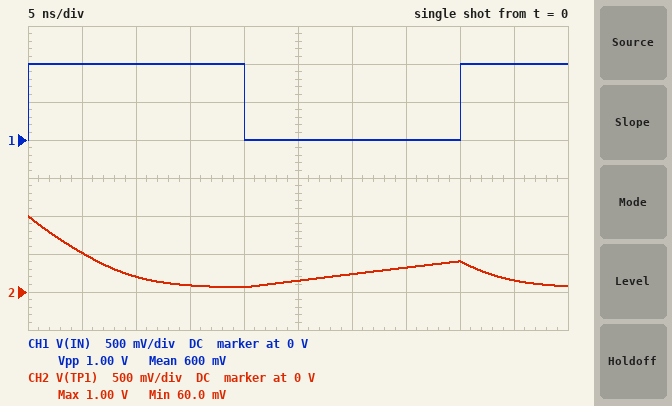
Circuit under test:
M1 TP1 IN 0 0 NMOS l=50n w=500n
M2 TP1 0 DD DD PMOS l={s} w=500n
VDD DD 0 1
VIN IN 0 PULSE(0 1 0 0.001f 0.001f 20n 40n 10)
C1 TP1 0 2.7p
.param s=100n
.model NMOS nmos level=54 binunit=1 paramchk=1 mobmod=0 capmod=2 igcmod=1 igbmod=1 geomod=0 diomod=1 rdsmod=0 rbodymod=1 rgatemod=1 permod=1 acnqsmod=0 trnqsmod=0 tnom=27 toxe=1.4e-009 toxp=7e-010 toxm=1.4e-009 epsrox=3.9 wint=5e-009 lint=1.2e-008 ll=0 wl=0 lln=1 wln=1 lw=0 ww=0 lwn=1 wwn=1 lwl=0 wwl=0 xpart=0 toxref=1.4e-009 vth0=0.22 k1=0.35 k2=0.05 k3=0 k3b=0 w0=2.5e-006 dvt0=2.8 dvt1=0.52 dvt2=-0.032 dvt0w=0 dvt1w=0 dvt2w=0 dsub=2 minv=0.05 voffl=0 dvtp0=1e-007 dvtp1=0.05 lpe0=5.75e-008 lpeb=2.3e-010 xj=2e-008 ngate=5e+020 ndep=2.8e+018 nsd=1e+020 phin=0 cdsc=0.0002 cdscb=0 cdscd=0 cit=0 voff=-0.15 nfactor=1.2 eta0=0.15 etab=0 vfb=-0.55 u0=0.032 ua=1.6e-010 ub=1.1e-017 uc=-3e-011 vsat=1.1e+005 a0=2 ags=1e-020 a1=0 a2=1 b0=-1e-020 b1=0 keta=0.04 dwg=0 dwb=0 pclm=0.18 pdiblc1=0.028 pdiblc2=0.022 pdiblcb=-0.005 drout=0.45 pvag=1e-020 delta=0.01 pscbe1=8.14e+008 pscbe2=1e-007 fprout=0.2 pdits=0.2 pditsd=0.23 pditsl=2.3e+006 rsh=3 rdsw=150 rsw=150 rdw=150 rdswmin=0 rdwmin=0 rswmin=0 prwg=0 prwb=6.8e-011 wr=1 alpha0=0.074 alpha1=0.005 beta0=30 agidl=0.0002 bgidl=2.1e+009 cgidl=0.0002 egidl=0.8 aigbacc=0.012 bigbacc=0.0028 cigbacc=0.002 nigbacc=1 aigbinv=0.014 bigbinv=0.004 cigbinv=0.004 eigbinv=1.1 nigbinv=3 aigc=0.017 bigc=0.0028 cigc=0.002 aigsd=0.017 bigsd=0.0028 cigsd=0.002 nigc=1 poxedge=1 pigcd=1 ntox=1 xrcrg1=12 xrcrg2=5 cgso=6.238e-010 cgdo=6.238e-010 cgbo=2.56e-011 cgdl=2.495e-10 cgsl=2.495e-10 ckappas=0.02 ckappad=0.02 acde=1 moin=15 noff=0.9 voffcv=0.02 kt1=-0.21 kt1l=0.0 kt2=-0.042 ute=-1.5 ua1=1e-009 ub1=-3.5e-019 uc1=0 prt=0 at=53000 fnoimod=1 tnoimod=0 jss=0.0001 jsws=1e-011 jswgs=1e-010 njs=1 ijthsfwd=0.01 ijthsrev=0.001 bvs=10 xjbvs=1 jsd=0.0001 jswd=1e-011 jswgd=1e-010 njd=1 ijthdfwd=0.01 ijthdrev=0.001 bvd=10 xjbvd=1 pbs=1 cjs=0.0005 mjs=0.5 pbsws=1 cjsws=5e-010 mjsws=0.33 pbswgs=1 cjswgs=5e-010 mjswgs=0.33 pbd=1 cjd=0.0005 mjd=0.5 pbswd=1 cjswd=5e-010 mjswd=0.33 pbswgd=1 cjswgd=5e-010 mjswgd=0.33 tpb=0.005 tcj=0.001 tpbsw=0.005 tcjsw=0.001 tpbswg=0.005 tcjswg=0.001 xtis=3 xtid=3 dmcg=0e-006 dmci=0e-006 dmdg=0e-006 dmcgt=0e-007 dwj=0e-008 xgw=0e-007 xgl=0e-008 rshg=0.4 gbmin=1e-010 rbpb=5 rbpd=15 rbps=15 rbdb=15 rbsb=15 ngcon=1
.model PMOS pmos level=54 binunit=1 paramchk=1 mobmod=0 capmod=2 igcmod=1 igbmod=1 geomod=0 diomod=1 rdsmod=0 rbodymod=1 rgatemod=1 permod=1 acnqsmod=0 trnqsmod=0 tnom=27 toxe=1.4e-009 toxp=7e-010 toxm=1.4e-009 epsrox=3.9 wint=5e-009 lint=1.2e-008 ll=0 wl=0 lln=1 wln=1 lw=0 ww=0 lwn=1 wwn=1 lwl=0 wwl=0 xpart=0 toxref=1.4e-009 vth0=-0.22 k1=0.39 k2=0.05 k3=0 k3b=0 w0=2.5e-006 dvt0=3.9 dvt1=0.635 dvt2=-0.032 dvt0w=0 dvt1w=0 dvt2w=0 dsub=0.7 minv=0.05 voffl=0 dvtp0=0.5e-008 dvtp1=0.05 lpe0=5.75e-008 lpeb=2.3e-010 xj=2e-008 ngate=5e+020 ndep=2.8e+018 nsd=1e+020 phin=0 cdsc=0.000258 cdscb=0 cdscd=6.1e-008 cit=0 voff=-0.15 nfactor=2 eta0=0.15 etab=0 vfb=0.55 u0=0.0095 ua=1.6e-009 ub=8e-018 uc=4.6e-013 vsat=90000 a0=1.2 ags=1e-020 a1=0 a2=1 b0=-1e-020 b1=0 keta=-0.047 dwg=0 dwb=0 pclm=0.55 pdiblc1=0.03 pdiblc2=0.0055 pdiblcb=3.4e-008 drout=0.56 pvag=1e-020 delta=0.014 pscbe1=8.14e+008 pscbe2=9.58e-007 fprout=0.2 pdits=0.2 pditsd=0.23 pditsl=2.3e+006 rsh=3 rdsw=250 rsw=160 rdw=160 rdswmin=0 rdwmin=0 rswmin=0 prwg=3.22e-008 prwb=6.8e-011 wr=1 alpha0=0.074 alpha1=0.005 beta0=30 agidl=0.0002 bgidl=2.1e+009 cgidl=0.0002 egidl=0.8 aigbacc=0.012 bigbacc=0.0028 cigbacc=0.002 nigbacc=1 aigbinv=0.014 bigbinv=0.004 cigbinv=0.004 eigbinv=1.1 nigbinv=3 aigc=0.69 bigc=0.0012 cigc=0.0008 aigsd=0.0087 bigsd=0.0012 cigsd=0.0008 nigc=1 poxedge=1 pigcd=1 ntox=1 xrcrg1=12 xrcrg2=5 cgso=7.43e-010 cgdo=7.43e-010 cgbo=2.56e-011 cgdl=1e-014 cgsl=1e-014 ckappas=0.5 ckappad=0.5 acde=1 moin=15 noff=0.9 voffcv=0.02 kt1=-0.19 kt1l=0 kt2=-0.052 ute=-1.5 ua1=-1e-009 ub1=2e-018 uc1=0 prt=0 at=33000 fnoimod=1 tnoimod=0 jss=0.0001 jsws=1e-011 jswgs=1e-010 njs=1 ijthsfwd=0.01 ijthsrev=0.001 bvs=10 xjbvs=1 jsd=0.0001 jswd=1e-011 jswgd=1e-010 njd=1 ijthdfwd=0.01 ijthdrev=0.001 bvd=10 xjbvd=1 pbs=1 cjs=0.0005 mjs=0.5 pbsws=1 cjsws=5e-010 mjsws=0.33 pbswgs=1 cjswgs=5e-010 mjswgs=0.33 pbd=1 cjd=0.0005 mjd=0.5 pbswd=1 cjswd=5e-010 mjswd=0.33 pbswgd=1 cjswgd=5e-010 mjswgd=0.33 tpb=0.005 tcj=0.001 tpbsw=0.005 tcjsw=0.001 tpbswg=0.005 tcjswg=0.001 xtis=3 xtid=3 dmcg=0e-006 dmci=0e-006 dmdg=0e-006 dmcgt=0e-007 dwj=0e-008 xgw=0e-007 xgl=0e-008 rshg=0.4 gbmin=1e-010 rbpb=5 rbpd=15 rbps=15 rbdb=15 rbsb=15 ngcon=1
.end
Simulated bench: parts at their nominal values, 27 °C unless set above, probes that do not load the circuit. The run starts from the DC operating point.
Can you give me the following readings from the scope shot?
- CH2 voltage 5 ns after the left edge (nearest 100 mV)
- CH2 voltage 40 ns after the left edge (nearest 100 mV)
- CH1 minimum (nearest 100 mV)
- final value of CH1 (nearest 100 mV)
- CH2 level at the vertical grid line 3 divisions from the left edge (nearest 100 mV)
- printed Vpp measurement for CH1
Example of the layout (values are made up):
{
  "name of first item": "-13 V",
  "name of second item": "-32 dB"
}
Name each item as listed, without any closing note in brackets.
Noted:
{
  "CH2 voltage 5 ns after the left edge": "500 mV",
  "CH2 voltage 40 ns after the left edge": "400 mV",
  "CH1 minimum": "0 V",
  "final value of CH1": "1.0 V",
  "CH2 level at the vertical grid line 3 divisions from the left edge": "100 mV",
  "printed Vpp measurement for CH1": "1.00 V"
}
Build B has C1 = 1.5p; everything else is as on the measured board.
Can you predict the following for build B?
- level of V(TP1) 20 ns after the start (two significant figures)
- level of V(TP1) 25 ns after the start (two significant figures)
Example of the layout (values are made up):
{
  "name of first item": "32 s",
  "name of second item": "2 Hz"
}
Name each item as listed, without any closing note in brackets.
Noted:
{
  "level of V(TP1) 20 ns after the start": "53 mV",
  "level of V(TP1) 25 ns after the start": "210 mV"
}
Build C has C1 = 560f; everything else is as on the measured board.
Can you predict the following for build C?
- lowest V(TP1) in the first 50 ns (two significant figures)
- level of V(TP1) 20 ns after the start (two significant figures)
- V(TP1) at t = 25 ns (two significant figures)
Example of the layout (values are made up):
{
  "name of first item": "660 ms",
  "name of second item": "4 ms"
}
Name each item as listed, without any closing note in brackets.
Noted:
{
  "lowest V(TP1) in the first 50 ns": "52 mV",
  "level of V(TP1) 20 ns after the start": "53 mV",
  "V(TP1) at t = 25 ns": "460 mV"
}
